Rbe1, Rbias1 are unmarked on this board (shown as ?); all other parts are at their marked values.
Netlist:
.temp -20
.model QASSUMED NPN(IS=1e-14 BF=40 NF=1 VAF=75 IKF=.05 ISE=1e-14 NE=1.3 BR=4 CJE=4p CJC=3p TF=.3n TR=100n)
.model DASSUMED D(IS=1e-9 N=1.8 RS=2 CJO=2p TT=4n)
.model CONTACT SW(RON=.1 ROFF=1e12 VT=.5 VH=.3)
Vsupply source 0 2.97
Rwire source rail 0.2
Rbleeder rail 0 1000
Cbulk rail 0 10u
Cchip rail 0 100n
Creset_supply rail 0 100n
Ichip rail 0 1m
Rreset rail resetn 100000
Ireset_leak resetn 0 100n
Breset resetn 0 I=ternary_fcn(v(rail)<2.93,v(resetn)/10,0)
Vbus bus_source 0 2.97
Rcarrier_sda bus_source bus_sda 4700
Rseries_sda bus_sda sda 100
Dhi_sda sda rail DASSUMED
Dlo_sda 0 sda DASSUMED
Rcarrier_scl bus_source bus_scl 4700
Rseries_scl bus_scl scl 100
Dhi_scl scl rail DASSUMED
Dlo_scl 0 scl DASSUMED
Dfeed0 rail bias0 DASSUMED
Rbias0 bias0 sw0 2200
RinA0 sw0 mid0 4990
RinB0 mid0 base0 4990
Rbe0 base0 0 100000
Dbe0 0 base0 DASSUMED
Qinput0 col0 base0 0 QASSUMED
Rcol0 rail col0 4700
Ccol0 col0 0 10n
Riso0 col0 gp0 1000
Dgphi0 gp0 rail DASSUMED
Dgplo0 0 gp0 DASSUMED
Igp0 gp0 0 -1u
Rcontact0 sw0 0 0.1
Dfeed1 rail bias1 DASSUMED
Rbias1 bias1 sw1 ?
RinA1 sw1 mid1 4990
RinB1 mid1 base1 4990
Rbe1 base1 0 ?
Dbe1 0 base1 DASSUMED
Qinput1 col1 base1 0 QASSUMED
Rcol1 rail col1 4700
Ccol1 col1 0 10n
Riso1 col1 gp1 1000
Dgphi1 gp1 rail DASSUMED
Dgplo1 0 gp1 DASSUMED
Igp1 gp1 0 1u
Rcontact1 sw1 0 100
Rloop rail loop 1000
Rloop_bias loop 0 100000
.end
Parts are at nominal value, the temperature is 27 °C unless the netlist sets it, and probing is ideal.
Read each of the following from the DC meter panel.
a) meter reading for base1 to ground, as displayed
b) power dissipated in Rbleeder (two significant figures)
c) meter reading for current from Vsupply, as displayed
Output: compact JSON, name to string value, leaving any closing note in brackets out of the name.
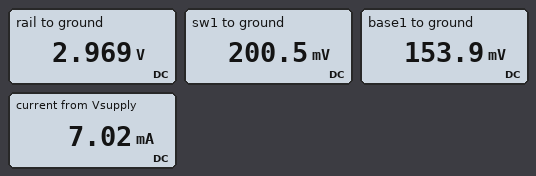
{"meter reading for base1 to ground, as displayed": "153.9 mV", "power dissipated in Rbleeder": "8.8 mW", "meter reading for current from Vsupply, as displayed": "7.02 mA"}
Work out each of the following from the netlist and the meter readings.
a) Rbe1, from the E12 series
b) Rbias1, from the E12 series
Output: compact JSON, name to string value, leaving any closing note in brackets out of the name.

{"Rbe1, from the E12 series": "33 kΩ", "Rbias1, from the E12 series": "1 kΩ"}
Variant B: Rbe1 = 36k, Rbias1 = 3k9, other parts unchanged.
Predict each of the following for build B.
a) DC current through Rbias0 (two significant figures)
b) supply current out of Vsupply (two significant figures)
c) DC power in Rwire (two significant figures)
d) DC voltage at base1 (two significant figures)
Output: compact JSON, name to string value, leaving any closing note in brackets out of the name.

{"DC current through Rbias0": "1.0 mA", "supply current out of Vsupply": "5.6 mA", "DC power in Rwire": "6.2 µW", "DC voltage at base1": "44 mV"}
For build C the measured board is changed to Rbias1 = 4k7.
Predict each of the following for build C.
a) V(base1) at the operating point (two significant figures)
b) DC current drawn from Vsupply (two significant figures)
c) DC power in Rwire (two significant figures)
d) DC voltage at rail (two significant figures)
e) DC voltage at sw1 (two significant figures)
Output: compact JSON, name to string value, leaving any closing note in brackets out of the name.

{"V(base1) at the operating point": "36 mV", "DC current drawn from Vsupply": "5.5 mA", "DC power in Rwire": "6.0 µW", "DC voltage at rail": "3.0 V", "DC voltage at sw1": "47 mV"}
